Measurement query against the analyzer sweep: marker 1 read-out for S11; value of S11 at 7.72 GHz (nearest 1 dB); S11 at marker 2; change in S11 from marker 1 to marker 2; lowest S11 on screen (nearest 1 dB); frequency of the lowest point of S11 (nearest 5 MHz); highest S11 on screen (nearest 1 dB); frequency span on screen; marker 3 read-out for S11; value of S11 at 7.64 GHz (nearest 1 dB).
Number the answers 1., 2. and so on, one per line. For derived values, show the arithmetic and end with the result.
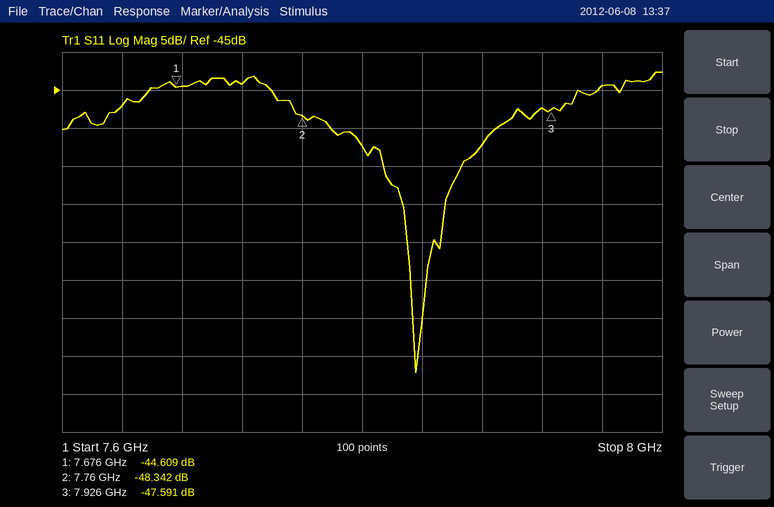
1. -44.609 dB
2. -44 dB
3. -48.342 dB
4. -48.342 − (-44.609) = -3.733 dB
5. -82 dB
6. 7.835 GHz
7. -43 dB
8. 400 MHz
9. -47.591 dB
10. -47 dB
